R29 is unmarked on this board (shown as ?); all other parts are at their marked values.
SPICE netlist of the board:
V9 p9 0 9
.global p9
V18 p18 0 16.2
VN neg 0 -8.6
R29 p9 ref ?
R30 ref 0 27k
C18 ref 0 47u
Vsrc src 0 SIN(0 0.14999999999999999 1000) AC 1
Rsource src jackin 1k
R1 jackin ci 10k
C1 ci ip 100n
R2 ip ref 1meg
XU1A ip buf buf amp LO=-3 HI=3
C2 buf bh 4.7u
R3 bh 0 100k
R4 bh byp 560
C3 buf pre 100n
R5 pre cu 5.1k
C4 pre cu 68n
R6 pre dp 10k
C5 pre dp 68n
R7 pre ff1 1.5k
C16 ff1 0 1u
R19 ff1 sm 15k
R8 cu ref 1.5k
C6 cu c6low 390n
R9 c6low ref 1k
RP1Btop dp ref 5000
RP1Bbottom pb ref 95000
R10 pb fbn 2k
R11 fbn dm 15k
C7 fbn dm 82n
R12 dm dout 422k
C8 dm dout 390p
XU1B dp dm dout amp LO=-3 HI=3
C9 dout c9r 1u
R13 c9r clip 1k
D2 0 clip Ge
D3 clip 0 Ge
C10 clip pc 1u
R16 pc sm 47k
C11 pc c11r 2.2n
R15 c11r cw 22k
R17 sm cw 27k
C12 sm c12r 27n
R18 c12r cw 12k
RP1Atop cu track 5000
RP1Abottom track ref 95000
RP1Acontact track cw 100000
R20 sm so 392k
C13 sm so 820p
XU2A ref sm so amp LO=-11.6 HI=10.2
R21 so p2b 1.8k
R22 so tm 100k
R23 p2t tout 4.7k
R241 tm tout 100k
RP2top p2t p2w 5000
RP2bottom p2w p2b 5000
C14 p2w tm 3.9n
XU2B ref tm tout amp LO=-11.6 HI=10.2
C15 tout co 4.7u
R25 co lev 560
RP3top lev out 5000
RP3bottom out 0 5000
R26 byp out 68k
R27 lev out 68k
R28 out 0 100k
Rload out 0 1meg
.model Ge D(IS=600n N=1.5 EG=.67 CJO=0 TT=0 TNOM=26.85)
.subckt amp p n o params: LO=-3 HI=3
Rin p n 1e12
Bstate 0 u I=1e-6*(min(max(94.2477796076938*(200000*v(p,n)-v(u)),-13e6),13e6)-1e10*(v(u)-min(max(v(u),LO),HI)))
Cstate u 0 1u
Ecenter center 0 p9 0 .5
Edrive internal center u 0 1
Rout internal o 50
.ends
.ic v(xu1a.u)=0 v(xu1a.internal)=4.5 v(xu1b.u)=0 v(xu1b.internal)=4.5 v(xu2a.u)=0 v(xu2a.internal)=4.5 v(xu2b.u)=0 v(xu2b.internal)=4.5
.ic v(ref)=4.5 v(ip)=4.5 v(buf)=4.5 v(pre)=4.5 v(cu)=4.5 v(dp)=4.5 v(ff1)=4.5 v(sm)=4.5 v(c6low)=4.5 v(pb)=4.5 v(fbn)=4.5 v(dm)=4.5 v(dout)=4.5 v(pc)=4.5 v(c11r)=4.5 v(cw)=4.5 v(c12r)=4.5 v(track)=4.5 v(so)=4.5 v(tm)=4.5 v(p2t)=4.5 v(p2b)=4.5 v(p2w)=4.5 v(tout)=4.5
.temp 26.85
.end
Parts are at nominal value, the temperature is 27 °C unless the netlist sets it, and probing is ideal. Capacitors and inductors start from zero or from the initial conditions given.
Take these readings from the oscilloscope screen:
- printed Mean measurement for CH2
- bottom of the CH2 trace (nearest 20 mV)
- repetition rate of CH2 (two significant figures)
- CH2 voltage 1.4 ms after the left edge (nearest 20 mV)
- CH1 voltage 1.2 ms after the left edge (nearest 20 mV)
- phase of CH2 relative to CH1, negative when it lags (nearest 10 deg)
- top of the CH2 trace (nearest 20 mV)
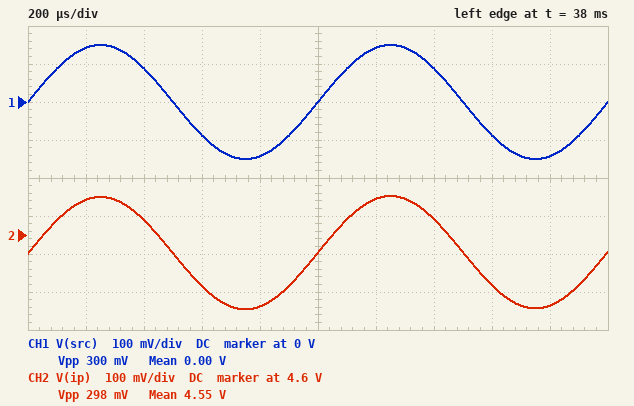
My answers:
4.55 V
4.40 V
1.0 kHz
4.64 V
140 mV
0 deg
4.70 V
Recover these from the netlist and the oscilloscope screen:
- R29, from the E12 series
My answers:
8.2 kΩ
